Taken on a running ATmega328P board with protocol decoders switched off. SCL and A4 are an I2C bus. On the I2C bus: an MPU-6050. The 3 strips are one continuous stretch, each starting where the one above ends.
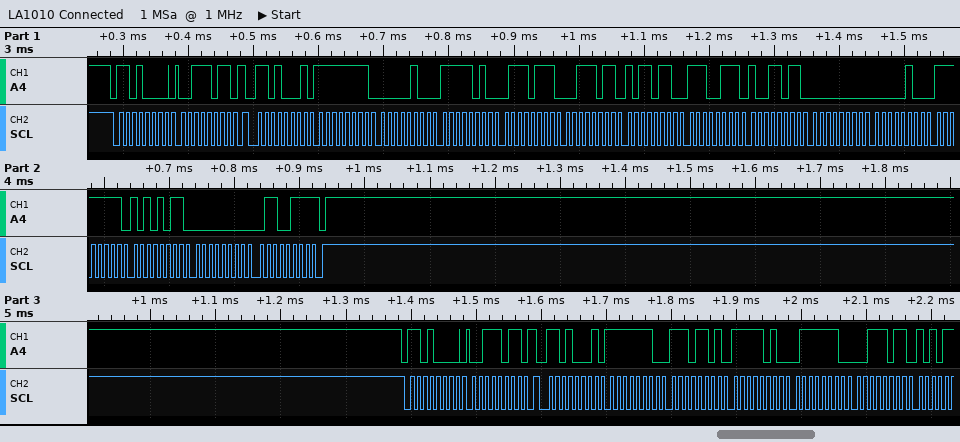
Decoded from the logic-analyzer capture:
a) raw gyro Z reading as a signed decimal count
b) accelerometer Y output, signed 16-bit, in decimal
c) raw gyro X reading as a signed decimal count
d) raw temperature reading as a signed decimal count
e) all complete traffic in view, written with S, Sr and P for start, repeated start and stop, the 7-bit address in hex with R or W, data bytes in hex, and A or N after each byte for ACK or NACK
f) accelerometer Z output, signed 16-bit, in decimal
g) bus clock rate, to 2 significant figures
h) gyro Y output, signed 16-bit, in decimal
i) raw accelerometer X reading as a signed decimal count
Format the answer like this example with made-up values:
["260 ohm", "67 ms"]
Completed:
["103", "-1417", "4", "-6245", "S 68W A 3B A Sr 68R A FF A 04 A FA A 77 A 3B A B6 A E7 A 9B A 00 A 04 A FF A AB A 00 A 67 N P S 68W A 3B A Sr 68R A FE A ED A FA A 7E A 3B A", "15286", "100 kHz", "-85", "-252"]
